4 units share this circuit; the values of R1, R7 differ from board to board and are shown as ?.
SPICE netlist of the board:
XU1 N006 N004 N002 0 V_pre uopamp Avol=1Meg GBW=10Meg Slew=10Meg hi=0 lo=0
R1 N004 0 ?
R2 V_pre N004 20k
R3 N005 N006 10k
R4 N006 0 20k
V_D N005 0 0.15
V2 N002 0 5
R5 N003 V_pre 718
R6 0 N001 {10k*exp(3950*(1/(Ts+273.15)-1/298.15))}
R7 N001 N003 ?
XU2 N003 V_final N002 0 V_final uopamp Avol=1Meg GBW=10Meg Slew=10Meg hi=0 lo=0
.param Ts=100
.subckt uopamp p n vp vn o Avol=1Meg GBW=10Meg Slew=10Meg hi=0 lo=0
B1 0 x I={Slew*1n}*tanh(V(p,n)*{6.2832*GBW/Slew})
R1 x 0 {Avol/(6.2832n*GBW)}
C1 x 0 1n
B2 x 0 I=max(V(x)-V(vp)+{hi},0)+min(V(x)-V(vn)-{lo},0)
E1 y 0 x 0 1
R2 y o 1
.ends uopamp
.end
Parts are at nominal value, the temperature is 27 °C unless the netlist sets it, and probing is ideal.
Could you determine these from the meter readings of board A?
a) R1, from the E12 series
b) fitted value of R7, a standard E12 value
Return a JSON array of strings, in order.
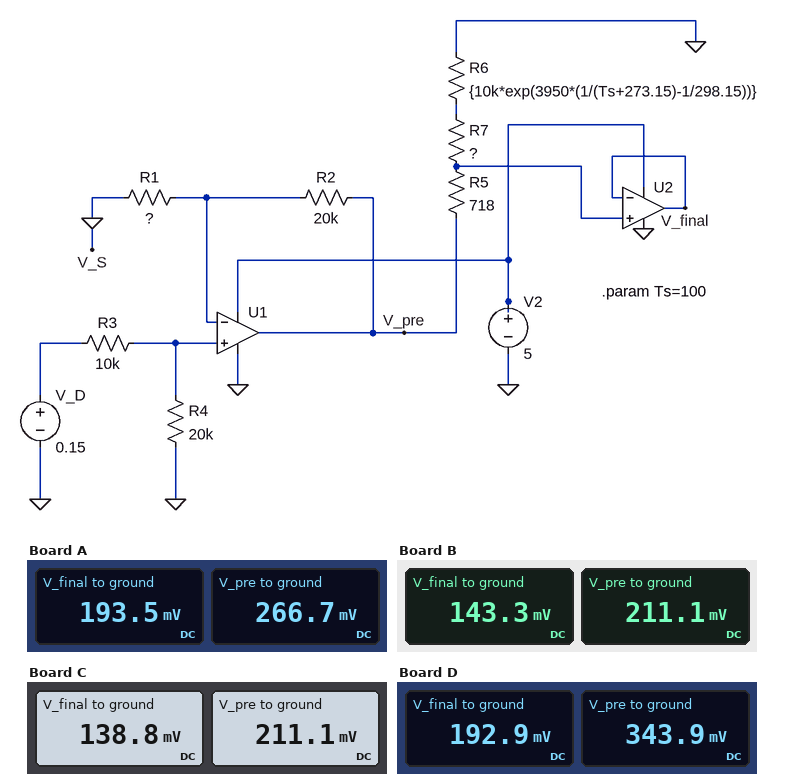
["12 kΩ", "1.2 kΩ"]
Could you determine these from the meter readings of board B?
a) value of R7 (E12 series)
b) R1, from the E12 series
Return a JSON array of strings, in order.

["820 Ω", "18 kΩ"]
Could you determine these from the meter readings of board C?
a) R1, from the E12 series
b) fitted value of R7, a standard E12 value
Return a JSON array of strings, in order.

["18 kΩ", "680 Ω"]
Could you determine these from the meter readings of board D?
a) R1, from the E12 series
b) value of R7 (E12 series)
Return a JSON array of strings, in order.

["8.2 kΩ", "220 Ω"]
